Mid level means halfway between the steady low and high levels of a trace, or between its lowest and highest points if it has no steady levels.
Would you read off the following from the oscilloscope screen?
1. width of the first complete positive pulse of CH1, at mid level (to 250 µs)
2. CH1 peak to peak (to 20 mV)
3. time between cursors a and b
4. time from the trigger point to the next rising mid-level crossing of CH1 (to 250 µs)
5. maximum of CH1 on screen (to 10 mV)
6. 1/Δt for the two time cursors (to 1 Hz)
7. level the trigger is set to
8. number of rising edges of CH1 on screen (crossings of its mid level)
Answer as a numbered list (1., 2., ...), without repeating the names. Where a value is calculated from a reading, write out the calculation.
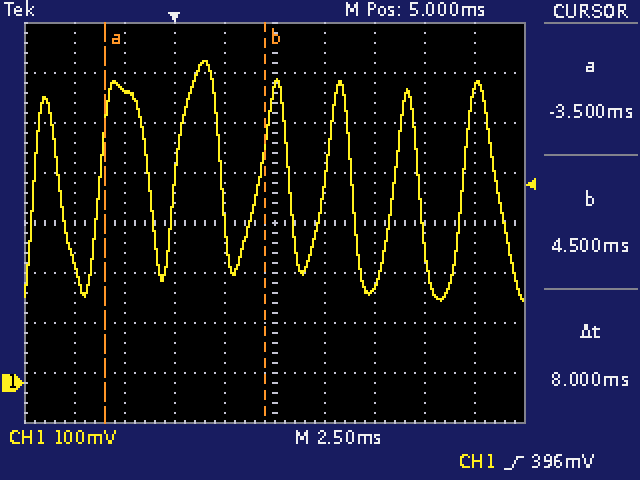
1. 1.25 ms
2. 480 mV
3. 8 ms
4. 4.25 ms
5. 640 mV
6. 1 / 8 ms ≈ 125 Hz
7. 396 mV
8. 7
